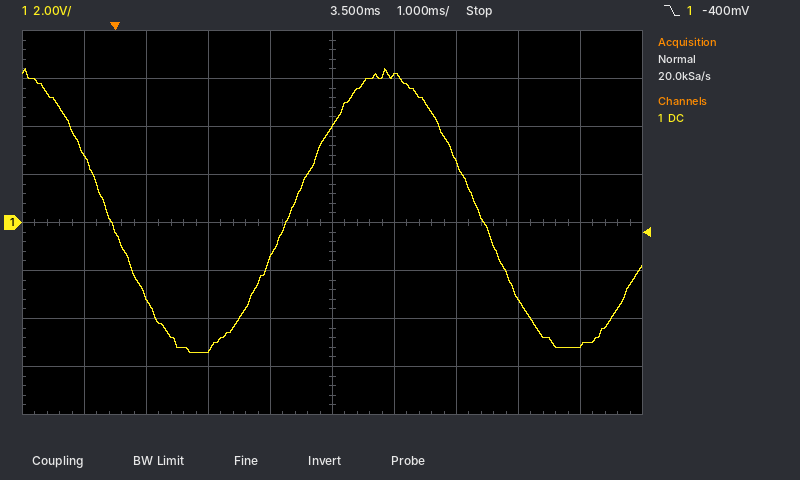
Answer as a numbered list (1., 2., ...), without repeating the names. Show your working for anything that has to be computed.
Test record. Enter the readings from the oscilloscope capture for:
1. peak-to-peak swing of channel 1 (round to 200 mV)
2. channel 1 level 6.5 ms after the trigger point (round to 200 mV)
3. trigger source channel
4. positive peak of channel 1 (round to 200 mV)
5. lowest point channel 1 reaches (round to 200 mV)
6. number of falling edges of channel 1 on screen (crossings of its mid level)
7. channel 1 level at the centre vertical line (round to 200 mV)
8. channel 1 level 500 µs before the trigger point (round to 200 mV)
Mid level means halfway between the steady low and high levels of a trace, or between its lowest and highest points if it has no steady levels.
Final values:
1. 6.4 V − (-5.4 V) = 11.8 V
2. -3.2 V
3. channel 1
4. 6.4 V
5. -5.4 V
6. 2
7. 4.0 V
8. 2.8 V
